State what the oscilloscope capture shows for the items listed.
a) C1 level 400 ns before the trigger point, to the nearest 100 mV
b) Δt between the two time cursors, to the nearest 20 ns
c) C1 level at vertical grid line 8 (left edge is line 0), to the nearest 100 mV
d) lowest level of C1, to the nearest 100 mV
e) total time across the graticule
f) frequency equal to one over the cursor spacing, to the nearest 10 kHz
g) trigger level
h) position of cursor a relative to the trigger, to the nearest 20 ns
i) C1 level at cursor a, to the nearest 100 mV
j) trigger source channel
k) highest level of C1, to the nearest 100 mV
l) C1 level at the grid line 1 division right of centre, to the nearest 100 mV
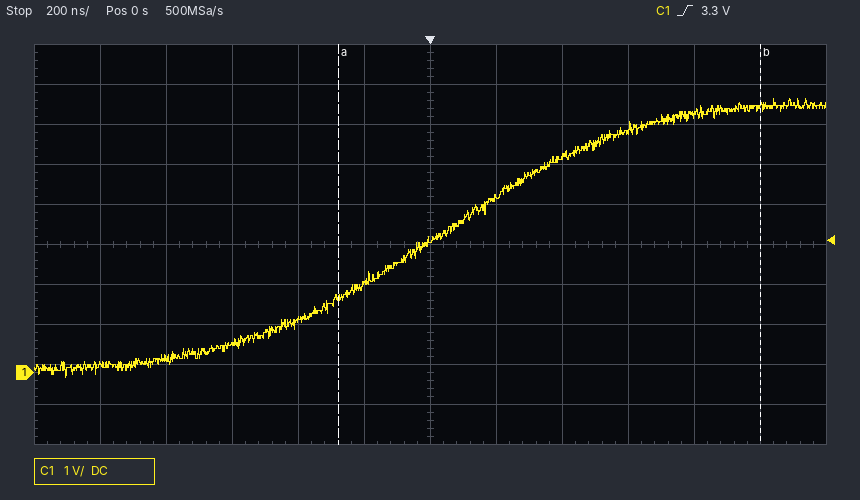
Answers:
1.3 V
1.28 µs
5.4 V
-100 mV
2.4 µs
780 kHz
3.3 V
-280 ns
1.9 V
C1
6.8 V
4.4 V
